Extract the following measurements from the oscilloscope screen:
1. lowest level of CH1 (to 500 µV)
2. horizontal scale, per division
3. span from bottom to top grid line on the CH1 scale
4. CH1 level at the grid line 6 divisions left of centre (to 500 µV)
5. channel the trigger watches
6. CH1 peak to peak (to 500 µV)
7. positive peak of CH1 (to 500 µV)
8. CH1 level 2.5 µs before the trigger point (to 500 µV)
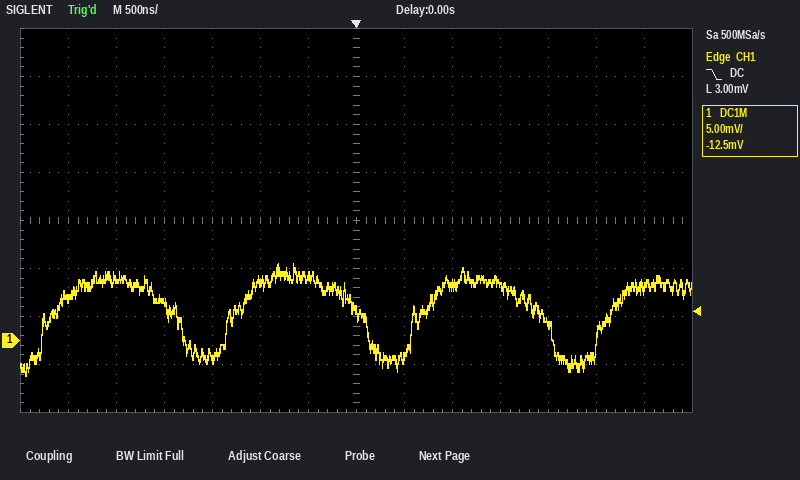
-3.5 mV
500 ns
40 mV
4.5 mV
CH1
11.5 mV
8.0 mV
6.5 mV
